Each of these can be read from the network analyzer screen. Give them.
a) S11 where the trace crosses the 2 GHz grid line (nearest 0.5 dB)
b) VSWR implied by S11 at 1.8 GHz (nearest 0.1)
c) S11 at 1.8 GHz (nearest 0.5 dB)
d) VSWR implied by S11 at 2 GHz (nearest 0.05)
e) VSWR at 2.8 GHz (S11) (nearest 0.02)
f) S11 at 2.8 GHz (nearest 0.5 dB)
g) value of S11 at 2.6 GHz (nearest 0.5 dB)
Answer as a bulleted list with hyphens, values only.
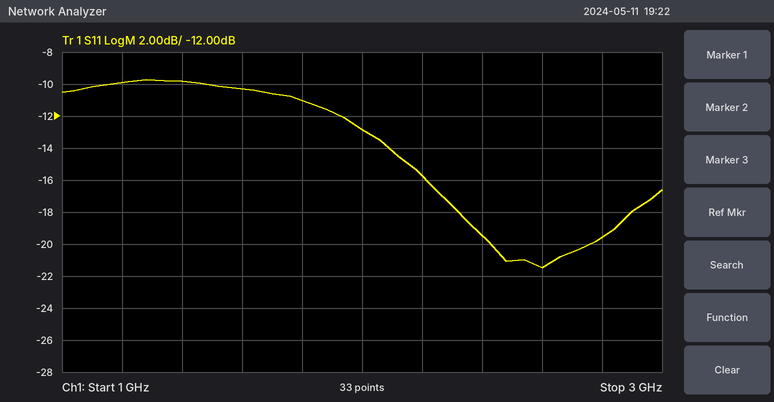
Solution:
- -13.0 dB
- 1.8
- -11.0 dB
- 1.60
- 1.24
- -19.5 dB
- -21.5 dB
